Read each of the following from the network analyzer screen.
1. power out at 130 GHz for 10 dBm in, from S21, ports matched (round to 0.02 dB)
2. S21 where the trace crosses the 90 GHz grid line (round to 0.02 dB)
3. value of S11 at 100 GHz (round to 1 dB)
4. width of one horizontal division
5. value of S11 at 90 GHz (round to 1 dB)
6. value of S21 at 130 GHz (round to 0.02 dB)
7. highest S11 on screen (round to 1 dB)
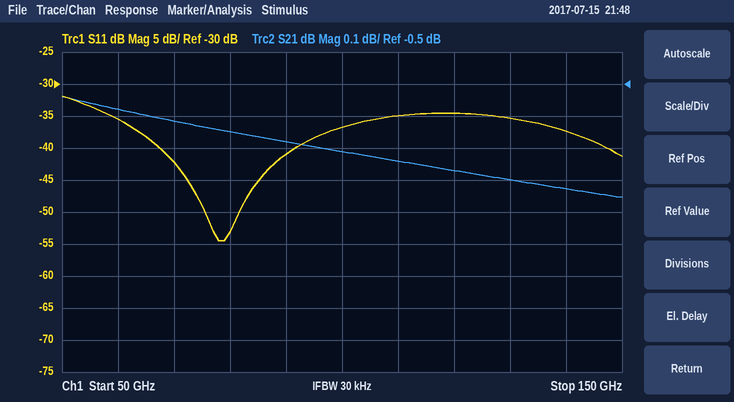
9.20 dBm
-0.68 dB
-37 dB
10 GHz
-41 dB
-0.80 dB
-32 dB
